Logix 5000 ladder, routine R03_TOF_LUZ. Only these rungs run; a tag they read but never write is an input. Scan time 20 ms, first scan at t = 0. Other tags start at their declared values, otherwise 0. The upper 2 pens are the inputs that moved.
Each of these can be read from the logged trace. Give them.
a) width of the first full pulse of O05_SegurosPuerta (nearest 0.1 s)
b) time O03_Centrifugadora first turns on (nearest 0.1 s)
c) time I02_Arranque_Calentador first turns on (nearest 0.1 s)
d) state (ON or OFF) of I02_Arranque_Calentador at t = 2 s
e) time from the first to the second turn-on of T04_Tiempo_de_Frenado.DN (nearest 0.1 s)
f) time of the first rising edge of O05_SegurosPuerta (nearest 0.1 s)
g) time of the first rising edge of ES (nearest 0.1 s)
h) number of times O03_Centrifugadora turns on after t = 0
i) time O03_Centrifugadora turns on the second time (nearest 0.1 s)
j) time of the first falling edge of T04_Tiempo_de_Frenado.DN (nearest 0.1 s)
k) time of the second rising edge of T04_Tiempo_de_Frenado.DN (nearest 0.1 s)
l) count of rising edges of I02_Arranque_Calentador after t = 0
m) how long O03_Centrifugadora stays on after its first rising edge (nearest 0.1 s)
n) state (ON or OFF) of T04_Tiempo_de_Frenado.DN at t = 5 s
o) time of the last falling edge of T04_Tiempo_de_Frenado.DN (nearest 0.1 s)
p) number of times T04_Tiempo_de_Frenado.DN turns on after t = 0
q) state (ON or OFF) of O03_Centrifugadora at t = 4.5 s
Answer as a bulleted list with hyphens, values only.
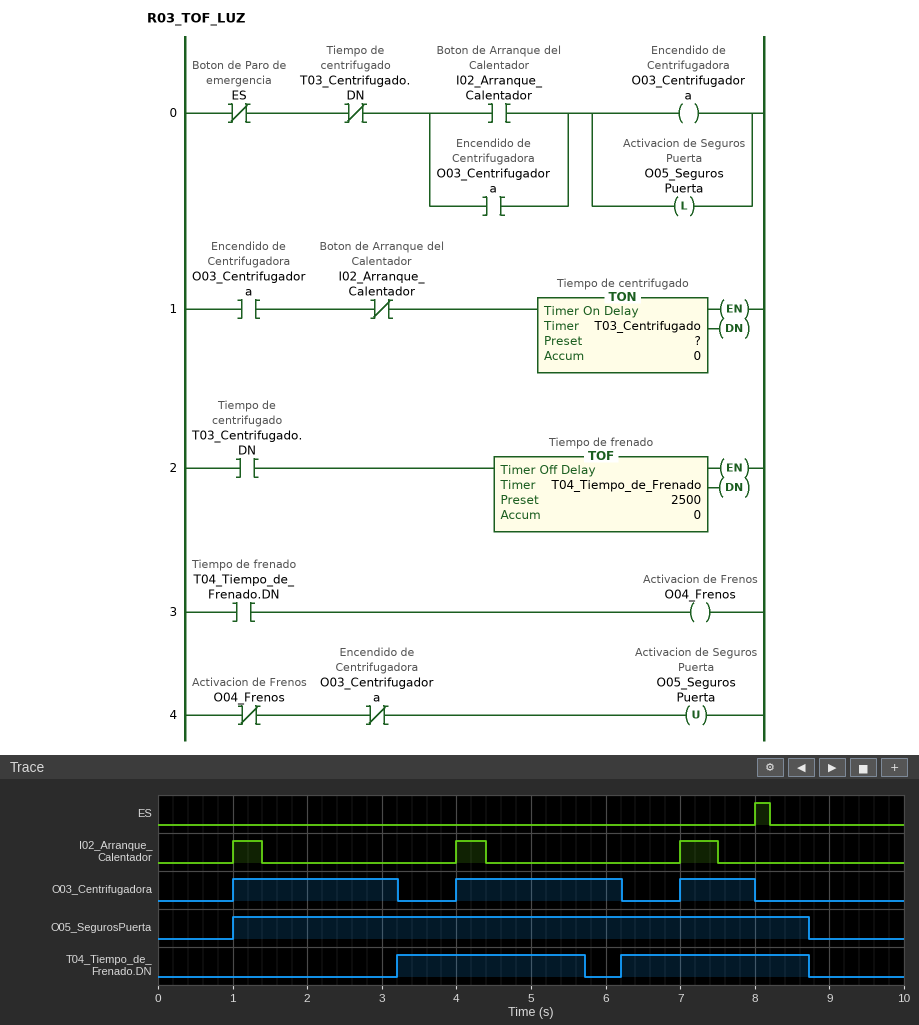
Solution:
- 7.7 s
- 1.0 s
- 1.0 s
- OFF
- 3.0 s
- 1.0 s
- 8.0 s
- 3
- 4.0 s
- 5.7 s
- 6.2 s
- 3
- 2.2 s
- ON
- 8.7 s
- 2
- ON
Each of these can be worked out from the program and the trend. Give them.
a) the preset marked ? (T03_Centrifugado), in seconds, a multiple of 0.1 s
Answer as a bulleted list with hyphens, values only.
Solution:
- 1.8 s
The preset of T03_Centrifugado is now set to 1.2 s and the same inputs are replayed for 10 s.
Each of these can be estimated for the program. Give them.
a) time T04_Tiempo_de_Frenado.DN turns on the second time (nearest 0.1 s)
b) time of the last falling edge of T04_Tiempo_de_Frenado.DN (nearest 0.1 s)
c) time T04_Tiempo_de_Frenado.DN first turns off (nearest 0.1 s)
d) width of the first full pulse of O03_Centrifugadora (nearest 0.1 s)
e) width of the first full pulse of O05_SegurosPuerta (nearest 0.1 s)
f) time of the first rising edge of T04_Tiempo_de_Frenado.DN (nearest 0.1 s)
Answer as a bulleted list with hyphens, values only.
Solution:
- 5.6 s
- 8.1 s
- 5.1 s
- 1.6 s
- 7.1 s
- 2.6 s
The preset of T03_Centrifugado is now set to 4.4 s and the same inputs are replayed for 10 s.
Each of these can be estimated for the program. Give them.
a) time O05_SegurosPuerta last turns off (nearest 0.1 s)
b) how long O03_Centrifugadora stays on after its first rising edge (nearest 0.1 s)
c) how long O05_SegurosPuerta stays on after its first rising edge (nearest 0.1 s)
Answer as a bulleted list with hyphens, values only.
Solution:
- 8.0 s
- 7.0 s
- 7.0 s
